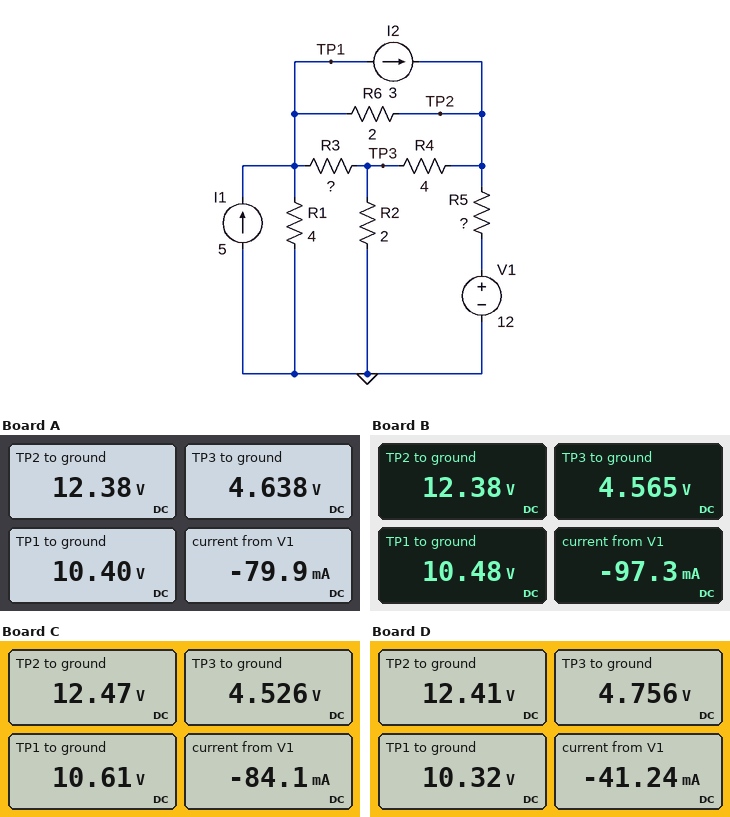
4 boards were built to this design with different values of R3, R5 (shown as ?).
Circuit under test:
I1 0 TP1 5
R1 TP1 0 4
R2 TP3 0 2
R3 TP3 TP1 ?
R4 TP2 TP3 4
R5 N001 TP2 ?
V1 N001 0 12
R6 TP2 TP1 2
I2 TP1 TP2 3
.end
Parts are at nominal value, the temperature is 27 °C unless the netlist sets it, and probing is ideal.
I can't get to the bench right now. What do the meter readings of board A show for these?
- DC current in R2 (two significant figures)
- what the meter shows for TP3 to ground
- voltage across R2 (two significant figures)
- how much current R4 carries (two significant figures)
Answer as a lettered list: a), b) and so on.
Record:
a) 2.3 A
b) 4.638 V
c) 4.6 V
d) 1.9 A
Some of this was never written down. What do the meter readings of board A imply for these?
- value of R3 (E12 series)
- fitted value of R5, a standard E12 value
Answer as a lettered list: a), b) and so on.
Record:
a) 15 Ω
b) 4.7 Ω
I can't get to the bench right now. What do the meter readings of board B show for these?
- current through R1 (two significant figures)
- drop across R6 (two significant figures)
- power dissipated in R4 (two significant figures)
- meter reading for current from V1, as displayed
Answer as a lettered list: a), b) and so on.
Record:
a) 2.6 A
b) 1.9 V
c) 15 W
d) -97.3 mA
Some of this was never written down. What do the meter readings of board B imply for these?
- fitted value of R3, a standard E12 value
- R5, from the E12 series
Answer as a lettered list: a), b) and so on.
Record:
a) 18 Ω
b) 3.9 Ω
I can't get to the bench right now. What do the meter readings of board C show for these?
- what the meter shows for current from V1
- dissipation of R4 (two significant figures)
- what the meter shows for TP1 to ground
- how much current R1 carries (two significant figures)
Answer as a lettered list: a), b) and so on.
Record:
a) -84.1 mA
b) 16 W
c) 10.61 V
d) 2.7 A
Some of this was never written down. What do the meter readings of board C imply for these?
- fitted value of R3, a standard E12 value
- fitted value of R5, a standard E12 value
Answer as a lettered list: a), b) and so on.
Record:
a) 22 Ω
b) 5.6 Ω
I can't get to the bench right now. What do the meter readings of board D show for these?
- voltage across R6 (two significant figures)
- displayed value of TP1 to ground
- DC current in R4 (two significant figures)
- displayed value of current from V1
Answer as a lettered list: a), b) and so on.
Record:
a) 2.1 V
b) 10.32 V
c) 1.9 A
d) -41.24 mA
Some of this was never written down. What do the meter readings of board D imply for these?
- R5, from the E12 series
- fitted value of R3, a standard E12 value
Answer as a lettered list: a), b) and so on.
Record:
a) 10 Ω
b) 12 Ω
